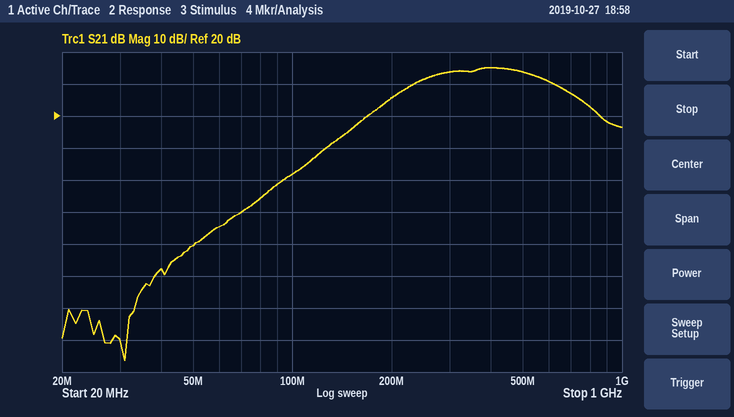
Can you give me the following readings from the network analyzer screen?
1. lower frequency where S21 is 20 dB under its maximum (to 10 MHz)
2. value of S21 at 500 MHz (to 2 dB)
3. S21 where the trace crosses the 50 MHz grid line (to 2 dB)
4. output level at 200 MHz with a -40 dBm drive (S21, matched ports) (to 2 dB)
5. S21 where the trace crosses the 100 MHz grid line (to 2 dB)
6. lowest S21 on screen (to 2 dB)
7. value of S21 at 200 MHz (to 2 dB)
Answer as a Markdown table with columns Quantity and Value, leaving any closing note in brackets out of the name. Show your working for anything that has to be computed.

| Quantity | Value |
|---|---|
| lower frequency where S21 is 20 dB under its maximum | 150 MHz |
| value of S21 at 500 MHz | 34 dB |
| S21 where the trace crosses the 50 MHz grid line | -20 dB |
| output level at 200 MHz with a -40 dBm drive (S21, matched ports) | -40 dBm + (26 dB) = -14 dBm |
| S21 where the trace crosses the 100 MHz grid line | 2 dB |
| lowest S21 on screen | -56 dB |
| value of S21 at 200 MHz | 26 dB |
